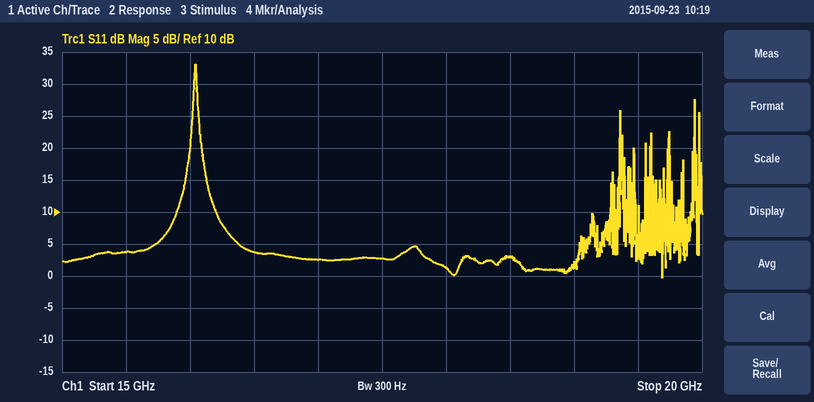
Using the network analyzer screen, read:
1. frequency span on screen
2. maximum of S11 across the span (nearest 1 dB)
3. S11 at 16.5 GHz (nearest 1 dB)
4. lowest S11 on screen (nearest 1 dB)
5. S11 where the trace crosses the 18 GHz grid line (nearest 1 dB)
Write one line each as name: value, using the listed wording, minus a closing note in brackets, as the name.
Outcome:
frequency span on screen: 5 GHz
maximum of S11 across the span: 33 dB
S11 at 16.5 GHz: 4 dB
lowest S11 on screen: 0 dB
S11 where the trace crosses the 18 GHz grid line: 1 dB
